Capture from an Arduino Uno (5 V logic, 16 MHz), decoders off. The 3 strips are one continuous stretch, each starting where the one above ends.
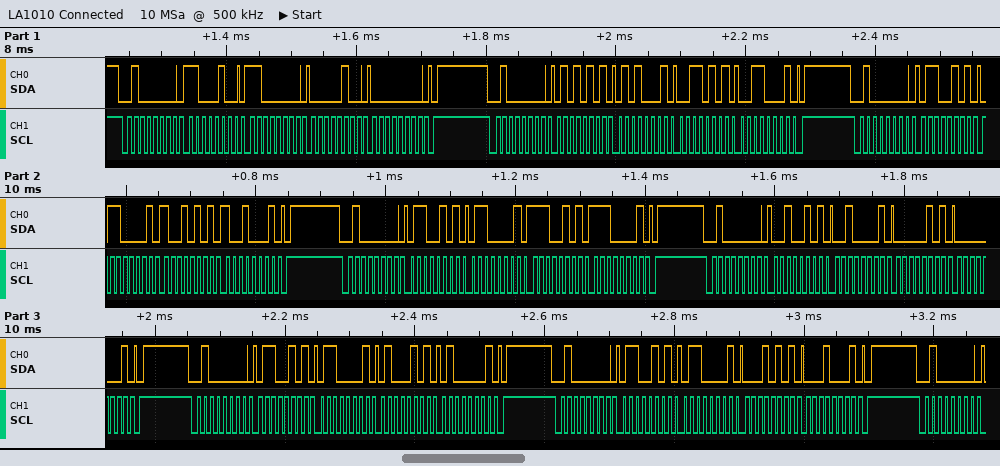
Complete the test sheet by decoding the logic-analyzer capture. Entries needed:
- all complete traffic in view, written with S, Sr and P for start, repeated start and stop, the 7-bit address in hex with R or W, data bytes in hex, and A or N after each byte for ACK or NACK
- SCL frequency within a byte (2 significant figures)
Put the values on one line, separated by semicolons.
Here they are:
S 20W A C4 A C0 A 04 A 00 A P S 20W A 55 A 51 A 35 A 31 A P S 20W A 65 A 61 A 95 A 91 A P S 20W A 65 A 61 A E5 A E1 A P S 20W A 25 A 21 A 05 A 01 A P S 20W A 65 A 61 A 45 A 41 A P S 20W A 65 A 61 A 15 A 11 A P S 20W A; 100 kHz
